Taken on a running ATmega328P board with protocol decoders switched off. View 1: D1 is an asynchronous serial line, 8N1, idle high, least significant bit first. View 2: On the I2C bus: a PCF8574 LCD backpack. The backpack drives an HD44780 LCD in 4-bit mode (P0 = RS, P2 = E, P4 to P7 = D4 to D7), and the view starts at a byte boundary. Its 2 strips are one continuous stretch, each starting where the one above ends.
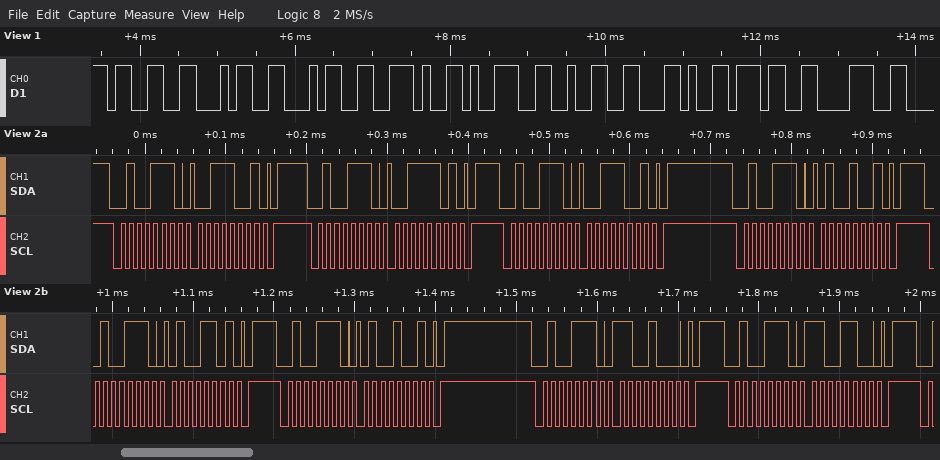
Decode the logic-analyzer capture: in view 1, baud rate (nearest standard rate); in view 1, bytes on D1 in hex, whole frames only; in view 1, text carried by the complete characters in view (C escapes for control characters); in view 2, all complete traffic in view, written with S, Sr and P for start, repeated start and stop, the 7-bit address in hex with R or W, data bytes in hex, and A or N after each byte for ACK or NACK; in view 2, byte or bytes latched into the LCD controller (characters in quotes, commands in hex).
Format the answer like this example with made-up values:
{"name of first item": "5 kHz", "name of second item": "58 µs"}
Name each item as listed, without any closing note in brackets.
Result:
{"in view 1, baud rate": "9600 baud", "in view 1, bytes on D1 in hex, whole frames only": "0x33 0x34 0x34 0x2E 0x39 0x32 0x2C 0x37 0x38", "in view 1, text carried by the complete characters in view": "\"344.92,78\"", "in view 2, all complete traffic in view, written with S, Sr and P for start, repeated start and stop, the 7-bit address in hex with R or W, data bytes in hex, and A or N after each byte for ACK or NACK": "S 27W A 39 A P S 27W A 3D A P S 27W A 39 A P S 27W A 49 A P S 27W A 4D A P S 27W A 49 A P S 27W A C8 A P S 27W A CC A P", "in view 2, byte or bytes latched into the LCD controller": "'4'"}
